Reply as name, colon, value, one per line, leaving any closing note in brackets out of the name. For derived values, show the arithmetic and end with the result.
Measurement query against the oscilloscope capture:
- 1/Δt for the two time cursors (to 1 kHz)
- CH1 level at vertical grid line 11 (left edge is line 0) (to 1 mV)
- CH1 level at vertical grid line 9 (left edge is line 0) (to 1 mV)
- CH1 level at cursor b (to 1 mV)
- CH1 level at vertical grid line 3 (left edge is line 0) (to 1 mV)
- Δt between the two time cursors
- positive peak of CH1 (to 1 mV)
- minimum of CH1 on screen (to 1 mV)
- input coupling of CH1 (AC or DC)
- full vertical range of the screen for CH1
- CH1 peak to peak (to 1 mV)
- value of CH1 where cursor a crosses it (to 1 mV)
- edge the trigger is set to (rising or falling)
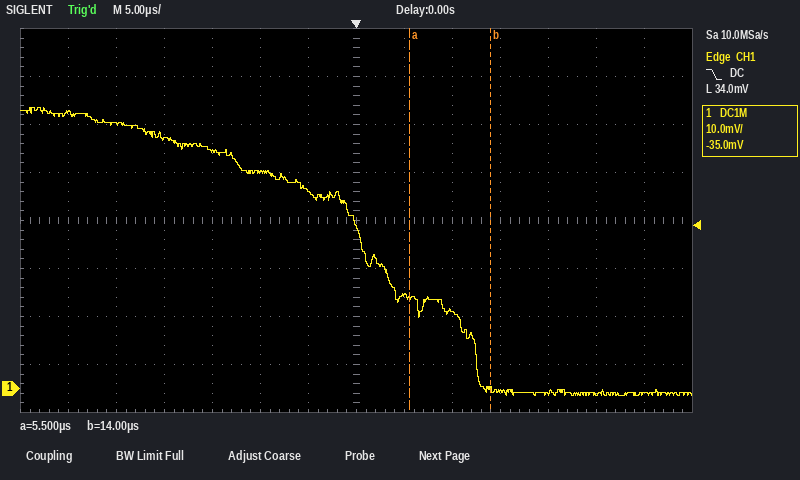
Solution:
1/Δt for the two time cursors: 1 / 8.5 µs ≈ 118 kHz
CH1 level at vertical grid line 11 (left edge is line 0): -1 mV
CH1 level at vertical grid line 9 (left edge is line 0): 16 mV
CH1 level at cursor b: 0 mV
CH1 level at vertical grid line 3 (left edge is line 0): 52 mV
Δt between the two time cursors: 14 µs − (5.5 µs) = 8.5 µs
positive peak of CH1: 59 mV
minimum of CH1 on screen: -1 mV
input coupling of CH1: DC
full vertical range of the screen for CH1: 80 mV
CH1 peak to peak: 59 mV − (-1 mV) = 60 mV
value of CH1 where cursor a crosses it: 19 mV
edge the trigger is set to: falling
